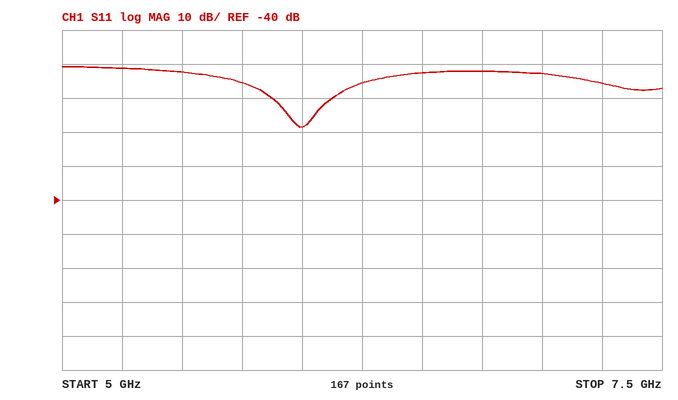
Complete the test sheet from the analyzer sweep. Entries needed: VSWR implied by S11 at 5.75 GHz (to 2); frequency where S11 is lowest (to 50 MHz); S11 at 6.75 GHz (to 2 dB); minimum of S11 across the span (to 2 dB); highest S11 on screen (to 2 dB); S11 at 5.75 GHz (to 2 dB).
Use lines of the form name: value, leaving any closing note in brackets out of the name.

VSWR implied by S11 at 5.75 GHz: 4
frequency where S11 is lowest: 6.00 GHz
S11 at 6.75 GHz: -2 dB
minimum of S11 across the span: -18 dB
highest S11 on screen: 0 dB
S11 at 5.75 GHz: -6 dB
